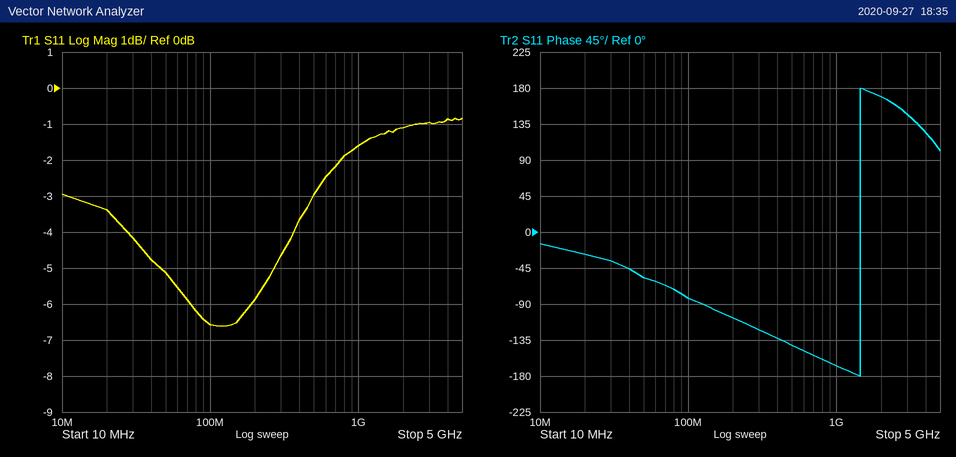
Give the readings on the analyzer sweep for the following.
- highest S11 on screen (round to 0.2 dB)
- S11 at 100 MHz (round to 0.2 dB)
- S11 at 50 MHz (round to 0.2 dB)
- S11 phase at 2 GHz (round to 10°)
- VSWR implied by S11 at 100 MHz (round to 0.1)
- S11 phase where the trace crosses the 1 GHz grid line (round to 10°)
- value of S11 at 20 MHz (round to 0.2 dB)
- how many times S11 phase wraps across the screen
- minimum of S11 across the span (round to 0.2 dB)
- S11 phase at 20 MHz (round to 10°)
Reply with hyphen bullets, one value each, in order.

- -0.8 dB
- -6.6 dB
- -5.2 dB
- 170°
- 2.8
- -170°
- -3.4 dB
- 1
- -6.6 dB
- -30°
